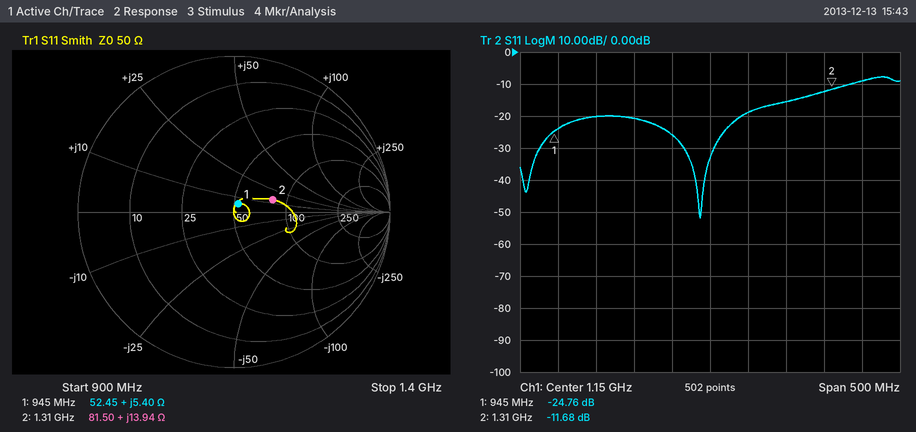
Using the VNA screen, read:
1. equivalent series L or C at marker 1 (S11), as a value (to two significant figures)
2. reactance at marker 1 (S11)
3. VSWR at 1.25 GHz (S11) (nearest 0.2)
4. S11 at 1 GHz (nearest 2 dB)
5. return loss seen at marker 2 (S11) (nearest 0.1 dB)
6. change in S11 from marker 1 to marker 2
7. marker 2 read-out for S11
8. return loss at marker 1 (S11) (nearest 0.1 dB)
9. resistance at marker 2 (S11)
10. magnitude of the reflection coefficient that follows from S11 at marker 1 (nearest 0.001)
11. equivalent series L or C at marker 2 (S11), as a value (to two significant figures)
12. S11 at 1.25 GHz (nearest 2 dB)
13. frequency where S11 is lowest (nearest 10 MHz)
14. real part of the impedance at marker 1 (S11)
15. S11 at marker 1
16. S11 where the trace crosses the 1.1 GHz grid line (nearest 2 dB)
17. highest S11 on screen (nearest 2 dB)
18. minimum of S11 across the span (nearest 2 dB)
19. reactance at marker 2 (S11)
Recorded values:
910 pH
+5.40 Ω
1.4
-20 dB
11.7 dB
13.08 dB
-11.68 dB
24.8 dB
81.50 Ω
0.058
1.7 nH
-16 dB
1.14 GHz
52.45 Ω
-24.76 dB
-26 dB
-8 dB
-52 dB
+13.94 Ω
